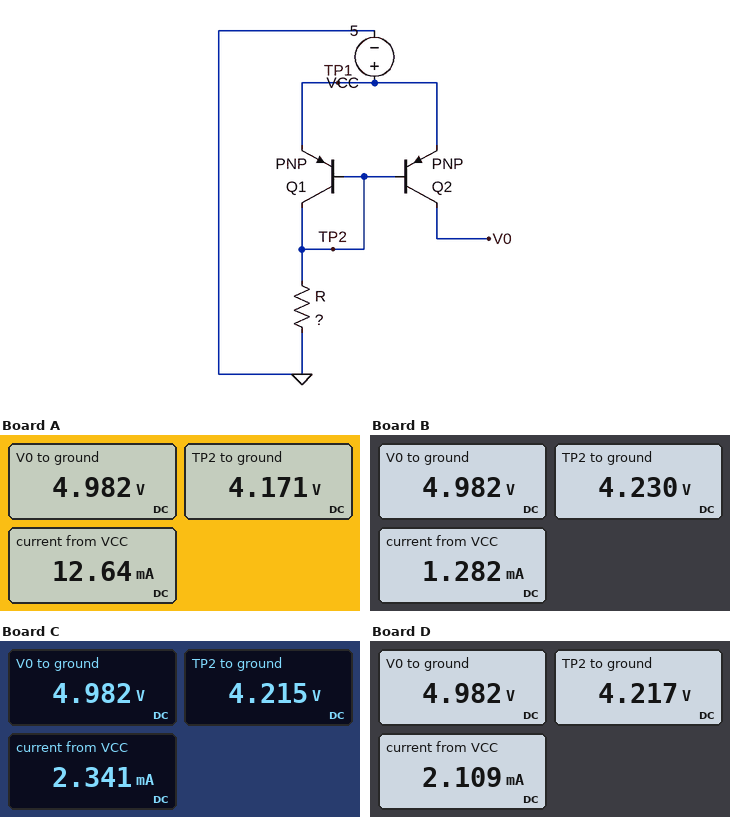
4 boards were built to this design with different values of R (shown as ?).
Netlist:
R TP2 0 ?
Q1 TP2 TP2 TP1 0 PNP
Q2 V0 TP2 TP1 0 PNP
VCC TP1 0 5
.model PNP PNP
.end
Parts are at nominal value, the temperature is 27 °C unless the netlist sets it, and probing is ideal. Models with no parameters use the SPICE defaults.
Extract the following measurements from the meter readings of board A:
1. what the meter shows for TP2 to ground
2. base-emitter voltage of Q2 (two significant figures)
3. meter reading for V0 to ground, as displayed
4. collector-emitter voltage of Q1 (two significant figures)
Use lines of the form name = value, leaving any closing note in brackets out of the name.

what the meter shows for TP2 to ground = 4.171 V
base-emitter voltage of Q2 = -830 mV
meter reading for V0 to ground, as displayed = 4.982 V
collector-emitter voltage of Q1 = -830 mV
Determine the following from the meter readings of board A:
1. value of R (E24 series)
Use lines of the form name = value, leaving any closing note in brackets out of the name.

value of R = 330 Ω
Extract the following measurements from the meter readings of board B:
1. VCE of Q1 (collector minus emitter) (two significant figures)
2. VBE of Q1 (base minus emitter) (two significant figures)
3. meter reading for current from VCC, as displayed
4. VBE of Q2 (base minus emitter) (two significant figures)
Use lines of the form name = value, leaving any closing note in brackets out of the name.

VCE of Q1 (collector minus emitter) = -770 mV
VBE of Q1 (base minus emitter) = -770 mV
meter reading for current from VCC, as displayed = 1.282 mA
VBE of Q2 (base minus emitter) = -770 mV
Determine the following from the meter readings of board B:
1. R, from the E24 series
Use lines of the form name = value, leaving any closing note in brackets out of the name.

R, from the E24 series = 3.3 kΩ
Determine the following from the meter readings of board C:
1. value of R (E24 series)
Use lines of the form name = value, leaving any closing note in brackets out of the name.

value of R = 1.8 kΩ
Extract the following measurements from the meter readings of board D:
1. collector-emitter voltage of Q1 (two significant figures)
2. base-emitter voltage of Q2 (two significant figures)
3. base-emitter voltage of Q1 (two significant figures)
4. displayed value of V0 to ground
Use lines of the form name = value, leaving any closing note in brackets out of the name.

collector-emitter voltage of Q1 = -780 mV
base-emitter voltage of Q2 = -780 mV
base-emitter voltage of Q1 = -780 mV
displayed value of V0 to ground = 4.982 V
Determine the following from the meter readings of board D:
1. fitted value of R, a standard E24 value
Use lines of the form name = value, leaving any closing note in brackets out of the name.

fitted value of R, a standard E24 value = 2 kΩ
